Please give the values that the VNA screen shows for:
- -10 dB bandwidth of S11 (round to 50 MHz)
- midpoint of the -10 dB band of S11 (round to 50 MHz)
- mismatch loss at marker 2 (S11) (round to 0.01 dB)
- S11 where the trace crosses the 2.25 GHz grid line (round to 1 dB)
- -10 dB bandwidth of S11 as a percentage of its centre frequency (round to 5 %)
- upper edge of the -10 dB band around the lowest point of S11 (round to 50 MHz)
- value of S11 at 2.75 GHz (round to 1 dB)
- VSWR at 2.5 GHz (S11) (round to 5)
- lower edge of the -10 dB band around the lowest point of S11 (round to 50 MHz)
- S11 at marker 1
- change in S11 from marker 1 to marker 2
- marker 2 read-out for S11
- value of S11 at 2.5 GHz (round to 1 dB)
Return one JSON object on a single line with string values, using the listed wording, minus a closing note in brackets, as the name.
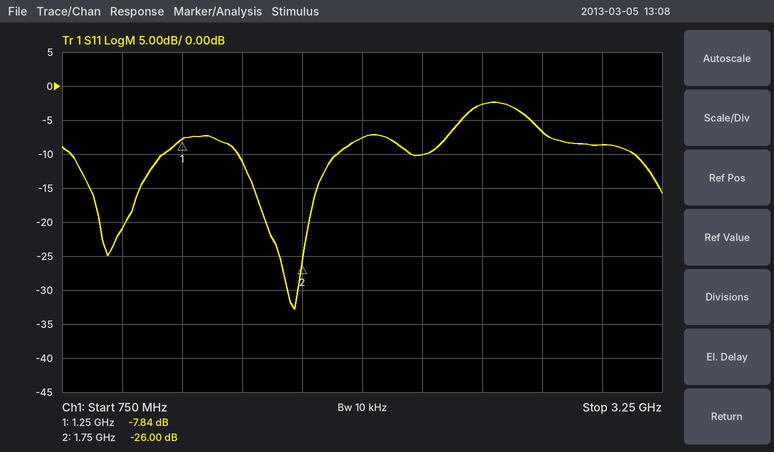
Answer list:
{"-10 dB bandwidth of S11": "400 MHz", "midpoint of the -10 dB band of S11": "1.70 GHz", "mismatch loss at marker 2 (S11)": "0.01 dB", "S11 where the trace crosses the 2.25 GHz grid line": "-10 dB", "-10 dB bandwidth of S11 as a percentage of its centre frequency": "25 %", "upper edge of the -10 dB band around the lowest point of S11": "1.90 GHz", "value of S11 at 2.75 GHz": "-7 dB", "VSWR at 2.5 GHz (S11)": "5", "lower edge of the -10 dB band around the lowest point of S11": "1.50 GHz", "S11 at marker 1": "-7.84 dB", "change in S11 from marker 1 to marker 2": "-18.16 dB", "marker 2 read-out for S11": "-26.00 dB", "value of S11 at 2.5 GHz": "-3 dB"}
